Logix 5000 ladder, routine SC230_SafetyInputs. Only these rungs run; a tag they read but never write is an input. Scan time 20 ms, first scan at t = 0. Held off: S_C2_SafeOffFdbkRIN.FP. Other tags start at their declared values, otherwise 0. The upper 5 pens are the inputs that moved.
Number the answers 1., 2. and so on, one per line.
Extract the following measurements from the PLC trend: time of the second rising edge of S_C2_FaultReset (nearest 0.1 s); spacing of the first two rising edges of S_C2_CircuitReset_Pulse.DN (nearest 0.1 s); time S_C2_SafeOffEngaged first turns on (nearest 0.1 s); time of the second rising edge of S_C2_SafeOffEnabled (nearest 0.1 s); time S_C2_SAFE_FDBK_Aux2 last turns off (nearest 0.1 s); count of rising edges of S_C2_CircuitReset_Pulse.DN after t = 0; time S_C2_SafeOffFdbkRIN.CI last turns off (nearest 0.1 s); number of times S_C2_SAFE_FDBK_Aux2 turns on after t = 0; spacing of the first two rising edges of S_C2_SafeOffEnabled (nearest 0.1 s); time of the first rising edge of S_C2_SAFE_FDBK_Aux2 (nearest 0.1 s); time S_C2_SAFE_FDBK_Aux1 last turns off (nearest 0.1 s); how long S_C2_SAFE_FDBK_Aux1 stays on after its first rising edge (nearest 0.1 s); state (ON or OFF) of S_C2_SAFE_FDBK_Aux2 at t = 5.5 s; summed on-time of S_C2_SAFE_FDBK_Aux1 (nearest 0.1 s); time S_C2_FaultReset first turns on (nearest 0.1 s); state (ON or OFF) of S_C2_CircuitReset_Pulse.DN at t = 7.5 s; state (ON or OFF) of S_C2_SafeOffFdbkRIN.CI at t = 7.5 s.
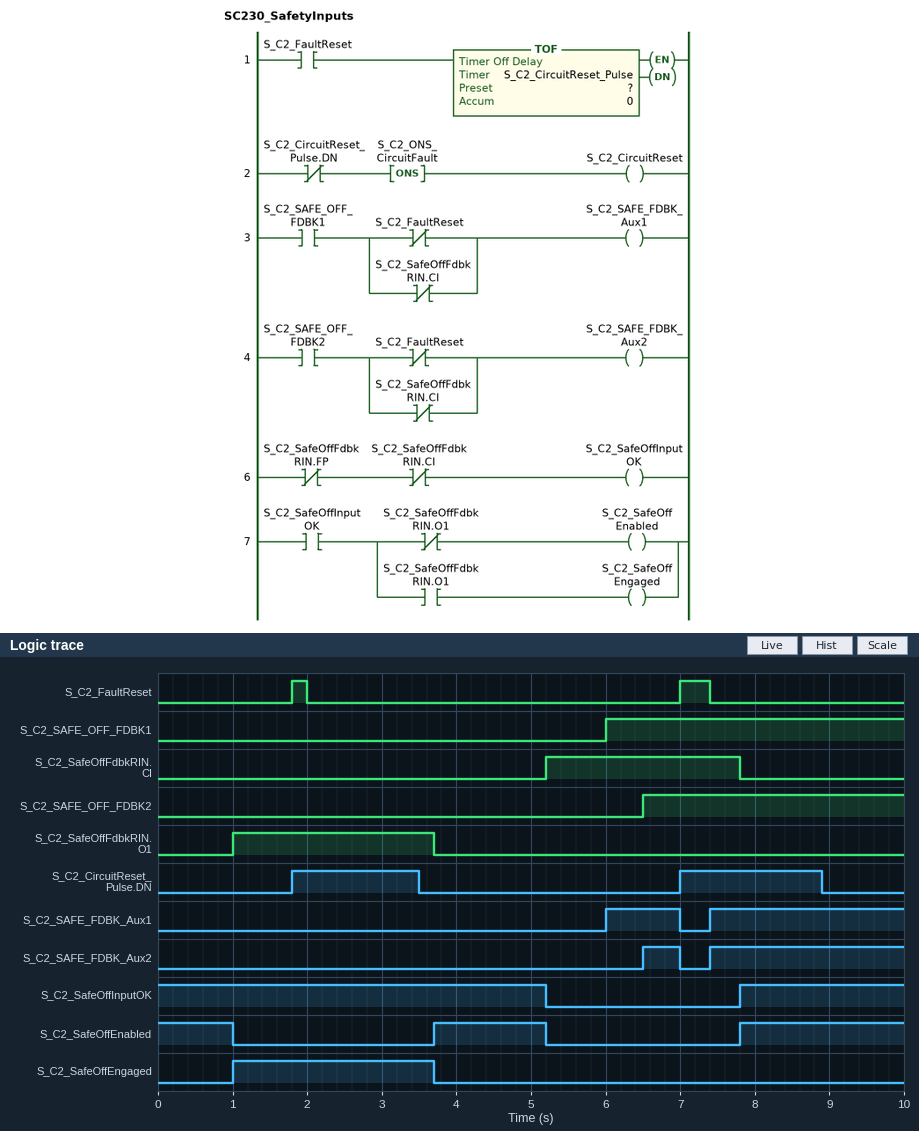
1. 7.0 s
2. 5.2 s
3. 1.0 s
4. 7.8 s
5. 7.0 s
6. 2
7. 7.8 s
8. 2
9. 4.1 s
10. 6.5 s
11. 7.0 s
12. 1.0 s
13. OFF
14. 3.6 s
15. 1.8 s
16. ON
17. ON
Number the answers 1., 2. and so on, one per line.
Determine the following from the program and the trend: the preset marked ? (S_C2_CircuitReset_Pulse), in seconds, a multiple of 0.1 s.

1. 1.5 s
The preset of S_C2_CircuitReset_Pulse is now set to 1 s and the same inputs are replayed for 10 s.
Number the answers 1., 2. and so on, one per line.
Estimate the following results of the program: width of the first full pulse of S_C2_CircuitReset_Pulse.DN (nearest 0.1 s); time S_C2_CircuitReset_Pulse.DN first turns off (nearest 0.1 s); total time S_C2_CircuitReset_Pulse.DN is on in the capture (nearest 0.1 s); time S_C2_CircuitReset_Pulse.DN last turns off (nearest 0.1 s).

1. 1.2 s
2. 3.0 s
3. 2.6 s
4. 8.4 s
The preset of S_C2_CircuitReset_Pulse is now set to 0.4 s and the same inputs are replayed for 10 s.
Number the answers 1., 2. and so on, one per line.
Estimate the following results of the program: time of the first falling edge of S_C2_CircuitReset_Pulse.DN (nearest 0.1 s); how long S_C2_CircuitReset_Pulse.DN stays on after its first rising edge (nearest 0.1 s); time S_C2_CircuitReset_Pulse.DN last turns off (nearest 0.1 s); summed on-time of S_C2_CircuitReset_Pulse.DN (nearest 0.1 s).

1. 2.4 s
2. 0.6 s
3. 7.8 s
4. 1.4 s
